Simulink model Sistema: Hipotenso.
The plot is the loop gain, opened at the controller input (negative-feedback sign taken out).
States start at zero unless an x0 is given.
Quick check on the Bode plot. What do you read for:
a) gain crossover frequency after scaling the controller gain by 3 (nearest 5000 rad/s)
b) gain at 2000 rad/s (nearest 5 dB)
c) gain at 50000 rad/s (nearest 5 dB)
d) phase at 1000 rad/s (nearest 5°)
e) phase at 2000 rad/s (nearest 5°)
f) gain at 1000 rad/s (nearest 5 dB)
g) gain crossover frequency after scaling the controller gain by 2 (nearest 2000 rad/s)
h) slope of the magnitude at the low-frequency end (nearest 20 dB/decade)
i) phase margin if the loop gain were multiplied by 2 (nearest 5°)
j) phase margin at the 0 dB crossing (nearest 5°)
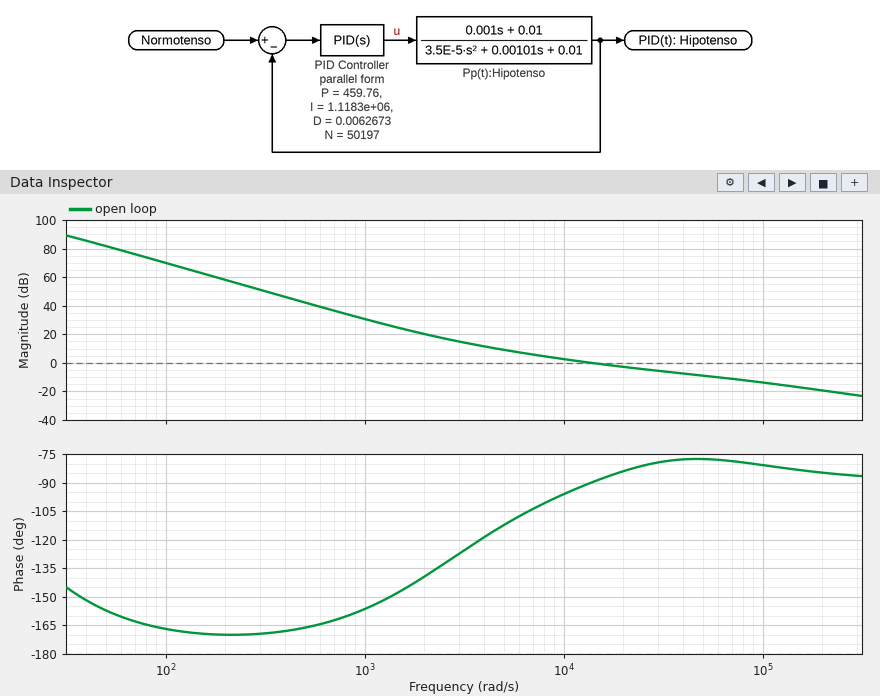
55000 rad/s
20 dB
-10 dB
-155°
-140°
30 dB
32000 rad/s
-40 dB/decade
100°
90°
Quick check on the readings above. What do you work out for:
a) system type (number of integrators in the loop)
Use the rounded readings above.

2
